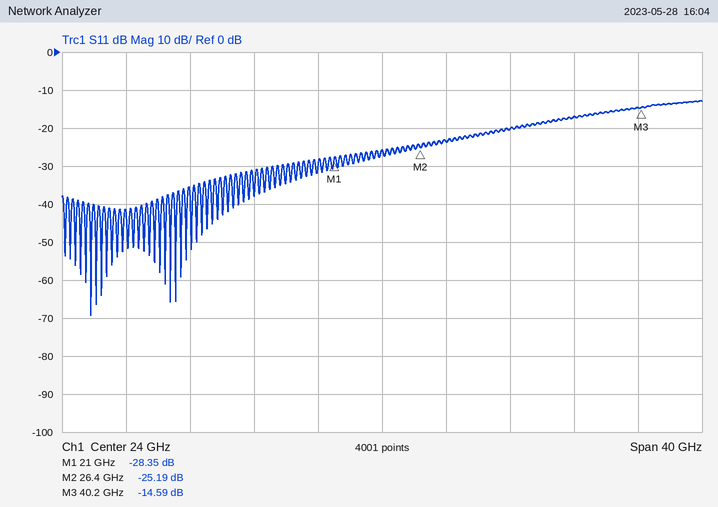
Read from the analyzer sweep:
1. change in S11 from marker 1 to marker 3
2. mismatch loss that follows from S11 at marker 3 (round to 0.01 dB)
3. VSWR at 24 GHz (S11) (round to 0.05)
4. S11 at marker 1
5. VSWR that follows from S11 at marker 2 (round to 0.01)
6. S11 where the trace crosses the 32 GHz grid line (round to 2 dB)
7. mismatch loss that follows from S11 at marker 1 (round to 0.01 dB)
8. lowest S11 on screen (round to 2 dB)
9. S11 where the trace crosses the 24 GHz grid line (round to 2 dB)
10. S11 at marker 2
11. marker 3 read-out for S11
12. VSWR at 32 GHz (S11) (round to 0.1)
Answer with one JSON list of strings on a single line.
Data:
["13.76 dB", "0.15 dB", "1.10", "-28.35 dB", "1.12", "-20 dB", "0.01 dB", "-70 dB", "-26 dB", "-25.19 dB", "-14.59 dB", "1.2"]
